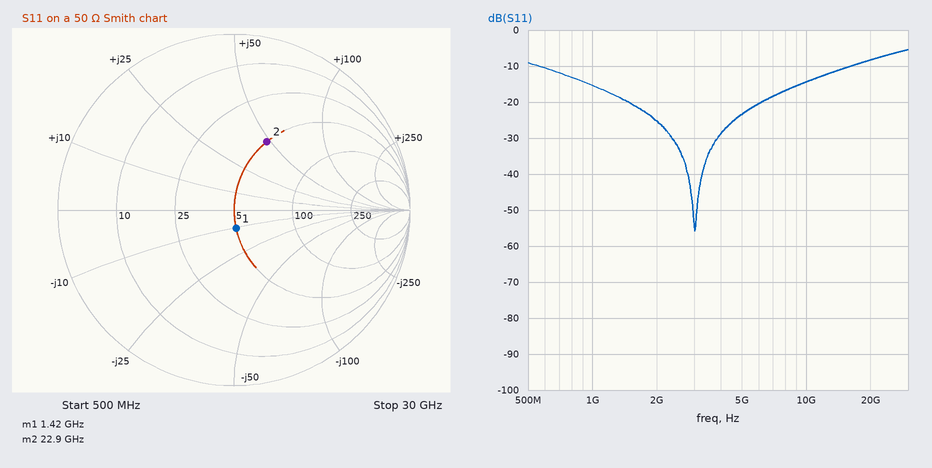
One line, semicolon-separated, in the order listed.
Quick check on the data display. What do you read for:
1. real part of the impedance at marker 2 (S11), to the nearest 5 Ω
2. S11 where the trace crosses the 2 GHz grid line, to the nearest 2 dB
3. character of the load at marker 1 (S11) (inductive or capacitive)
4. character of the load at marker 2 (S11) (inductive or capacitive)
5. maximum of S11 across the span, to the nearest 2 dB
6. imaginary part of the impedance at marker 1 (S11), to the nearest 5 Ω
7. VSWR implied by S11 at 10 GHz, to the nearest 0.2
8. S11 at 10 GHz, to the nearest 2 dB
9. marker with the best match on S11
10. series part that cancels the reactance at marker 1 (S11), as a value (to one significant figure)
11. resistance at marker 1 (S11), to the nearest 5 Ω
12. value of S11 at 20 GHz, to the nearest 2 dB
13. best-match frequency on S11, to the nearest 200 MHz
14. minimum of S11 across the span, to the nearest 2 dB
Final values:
50 Ω; -26 dB; capacitive; inductive; -6 dB; -10 Ω; 1.4; -14 dB; marker 1; 1 nH; 50 Ω; -8 dB; 3.0 GHz; -56 dB
